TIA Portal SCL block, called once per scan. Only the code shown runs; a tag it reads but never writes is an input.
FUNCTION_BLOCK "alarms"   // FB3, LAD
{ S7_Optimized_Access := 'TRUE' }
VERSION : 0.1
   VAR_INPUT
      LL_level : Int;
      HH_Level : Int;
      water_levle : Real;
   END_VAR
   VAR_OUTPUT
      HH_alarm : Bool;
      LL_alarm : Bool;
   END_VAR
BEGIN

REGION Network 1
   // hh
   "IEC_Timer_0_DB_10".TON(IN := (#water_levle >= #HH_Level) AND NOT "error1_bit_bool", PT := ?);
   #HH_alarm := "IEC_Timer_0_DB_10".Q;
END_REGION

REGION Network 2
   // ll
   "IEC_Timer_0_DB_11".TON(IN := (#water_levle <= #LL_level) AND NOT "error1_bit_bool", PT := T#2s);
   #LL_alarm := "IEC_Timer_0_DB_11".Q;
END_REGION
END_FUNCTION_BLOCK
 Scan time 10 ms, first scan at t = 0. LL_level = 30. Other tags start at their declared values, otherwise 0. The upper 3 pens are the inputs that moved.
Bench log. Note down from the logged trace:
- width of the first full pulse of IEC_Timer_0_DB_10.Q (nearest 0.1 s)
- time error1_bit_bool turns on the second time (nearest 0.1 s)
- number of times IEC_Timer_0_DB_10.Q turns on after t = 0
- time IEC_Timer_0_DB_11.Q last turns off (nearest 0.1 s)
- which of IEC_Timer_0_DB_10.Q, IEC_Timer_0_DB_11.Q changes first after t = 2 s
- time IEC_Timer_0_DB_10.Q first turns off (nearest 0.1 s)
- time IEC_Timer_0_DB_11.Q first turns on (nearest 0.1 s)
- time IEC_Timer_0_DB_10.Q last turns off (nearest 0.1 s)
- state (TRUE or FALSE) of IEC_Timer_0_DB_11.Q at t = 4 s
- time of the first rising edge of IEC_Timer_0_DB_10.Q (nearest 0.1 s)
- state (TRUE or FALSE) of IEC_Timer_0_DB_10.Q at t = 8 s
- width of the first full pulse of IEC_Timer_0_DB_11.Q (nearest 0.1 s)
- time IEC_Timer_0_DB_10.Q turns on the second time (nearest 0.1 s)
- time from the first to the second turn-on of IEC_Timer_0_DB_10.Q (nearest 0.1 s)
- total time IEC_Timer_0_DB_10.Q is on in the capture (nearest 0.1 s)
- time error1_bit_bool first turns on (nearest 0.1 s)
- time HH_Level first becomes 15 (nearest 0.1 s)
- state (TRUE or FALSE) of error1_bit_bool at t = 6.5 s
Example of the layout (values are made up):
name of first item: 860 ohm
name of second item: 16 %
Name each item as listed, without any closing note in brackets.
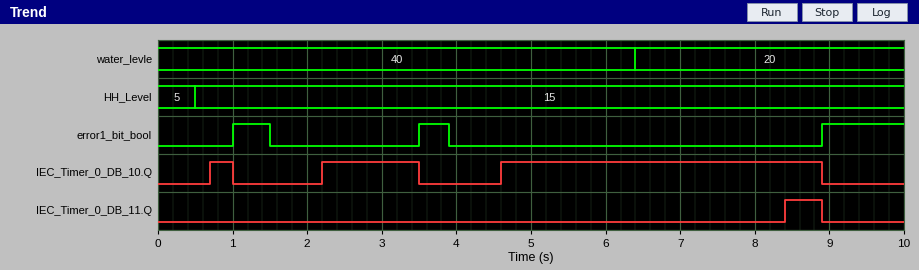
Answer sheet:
width of the first full pulse of IEC_Timer_0_DB_10.Q: 0.3 s
time error1_bit_bool turns on the second time: 3.5 s
number of times IEC_Timer_0_DB_10.Q turns on after t = 0: 3
time IEC_Timer_0_DB_11.Q last turns off: 8.9 s
which of IEC_Timer_0_DB_10.Q, IEC_Timer_0_DB_11.Q changes first after t = 2 s: IEC_Timer_0_DB_10.Q
time IEC_Timer_0_DB_10.Q first turns off: 1.0 s
time IEC_Timer_0_DB_11.Q first turns on: 8.4 s
time IEC_Timer_0_DB_10.Q last turns off: 8.9 s
state (TRUE or FALSE) of IEC_Timer_0_DB_11.Q at t = 4 s: FALSE
time of the first rising edge of IEC_Timer_0_DB_10.Q: 0.7 s
state (TRUE or FALSE) of IEC_Timer_0_DB_10.Q at t = 8 s: TRUE
width of the first full pulse of IEC_Timer_0_DB_11.Q: 0.5 s
time IEC_Timer_0_DB_10.Q turns on the second time: 2.2 s
time from the first to the second turn-on of IEC_Timer_0_DB_10.Q: 1.5 s
total time IEC_Timer_0_DB_10.Q is on in the capture: 5.9 s
time error1_bit_bool first turns on: 1.0 s
time HH_Level first becomes 15: 0.5 s
state (TRUE or FALSE) of error1_bit_bool at t = 6.5 s: FALSE
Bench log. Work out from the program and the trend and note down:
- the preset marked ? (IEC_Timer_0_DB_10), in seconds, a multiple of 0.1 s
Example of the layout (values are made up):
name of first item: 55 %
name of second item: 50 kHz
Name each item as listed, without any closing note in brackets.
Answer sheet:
the preset marked ? (IEC_Timer_0_DB_10), in seconds, a multiple of 0.1 s: 0.7 s
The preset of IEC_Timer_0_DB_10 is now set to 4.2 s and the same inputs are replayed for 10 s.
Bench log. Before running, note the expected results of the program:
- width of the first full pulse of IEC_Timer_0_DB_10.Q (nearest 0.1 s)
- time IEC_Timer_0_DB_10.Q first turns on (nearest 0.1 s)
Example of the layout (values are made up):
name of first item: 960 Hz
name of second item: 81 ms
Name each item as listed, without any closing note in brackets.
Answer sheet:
width of the first full pulse of IEC_Timer_0_DB_10.Q: 0.8 s
time IEC_Timer_0_DB_10.Q first turns on: 8.1 s
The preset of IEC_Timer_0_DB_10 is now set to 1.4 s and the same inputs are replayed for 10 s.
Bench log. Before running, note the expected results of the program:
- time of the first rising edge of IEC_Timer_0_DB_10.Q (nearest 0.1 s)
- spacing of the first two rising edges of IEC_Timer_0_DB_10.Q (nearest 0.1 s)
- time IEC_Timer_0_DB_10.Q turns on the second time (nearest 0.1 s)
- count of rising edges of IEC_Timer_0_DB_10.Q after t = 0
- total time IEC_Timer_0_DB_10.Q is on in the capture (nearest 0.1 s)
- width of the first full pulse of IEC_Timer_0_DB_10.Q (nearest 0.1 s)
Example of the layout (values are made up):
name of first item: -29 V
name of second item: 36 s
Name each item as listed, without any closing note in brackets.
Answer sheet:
time of the first rising edge of IEC_Timer_0_DB_10.Q: 2.9 s
spacing of the first two rising edges of IEC_Timer_0_DB_10.Q: 2.4 s
time IEC_Timer_0_DB_10.Q turns on the second time: 5.3 s
count of rising edges of IEC_Timer_0_DB_10.Q after t = 0: 2
total time IEC_Timer_0_DB_10.Q is on in the capture: 4.2 s
width of the first full pulse of IEC_Timer_0_DB_10.Q: 0.6 s
